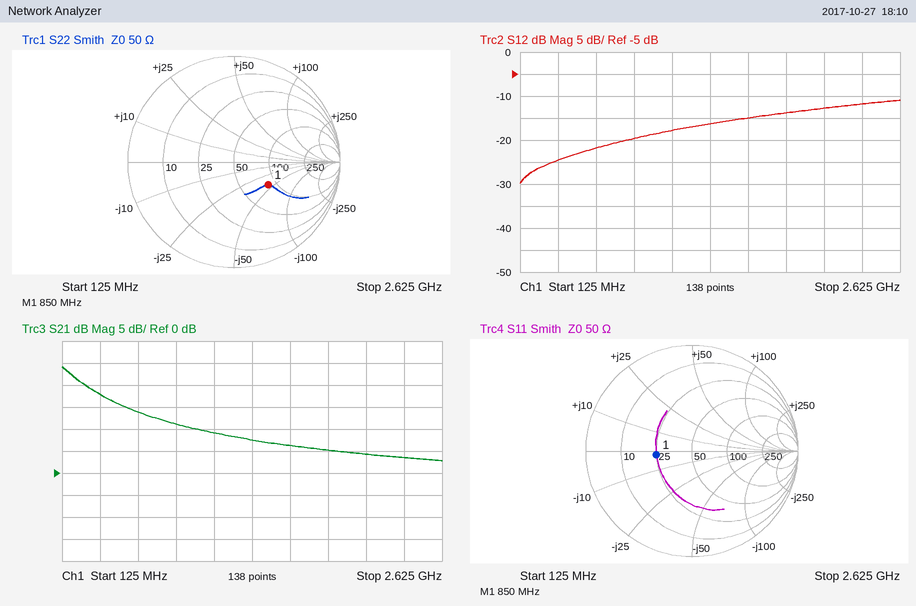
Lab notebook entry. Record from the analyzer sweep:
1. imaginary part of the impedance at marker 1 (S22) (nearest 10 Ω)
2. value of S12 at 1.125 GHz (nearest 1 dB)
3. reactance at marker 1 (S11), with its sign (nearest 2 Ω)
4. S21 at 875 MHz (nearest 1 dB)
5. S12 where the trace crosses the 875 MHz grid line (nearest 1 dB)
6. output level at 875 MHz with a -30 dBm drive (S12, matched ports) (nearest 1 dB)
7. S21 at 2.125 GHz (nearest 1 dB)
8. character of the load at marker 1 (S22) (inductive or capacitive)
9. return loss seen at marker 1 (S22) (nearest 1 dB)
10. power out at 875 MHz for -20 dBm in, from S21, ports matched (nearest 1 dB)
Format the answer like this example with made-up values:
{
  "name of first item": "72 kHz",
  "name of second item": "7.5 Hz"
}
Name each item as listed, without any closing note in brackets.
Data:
{
  "imaginary part of the impedance at marker 1 (S22)": "-40 Ω",
  "value of S12 at 1.125 GHz": "-18 dB",
  "reactance at marker 1 (S11), with its sign": "-2 Ω",
  "S21 at 875 MHz": "11 dB",
  "S12 where the trace crosses the 875 MHz grid line": "-20 dB",
  "output level at 875 MHz with a -30 dBm drive (S12, matched ports)": "-50 dBm",
  "S21 at 2.125 GHz": "4 dB",
  "character of the load at marker 1 (S22)": "capacitive",
  "return loss seen at marker 1 (S22)": "8 dB",
  "power out at 875 MHz for -20 dBm in, from S21, ports matched": "-9 dBm"
}
